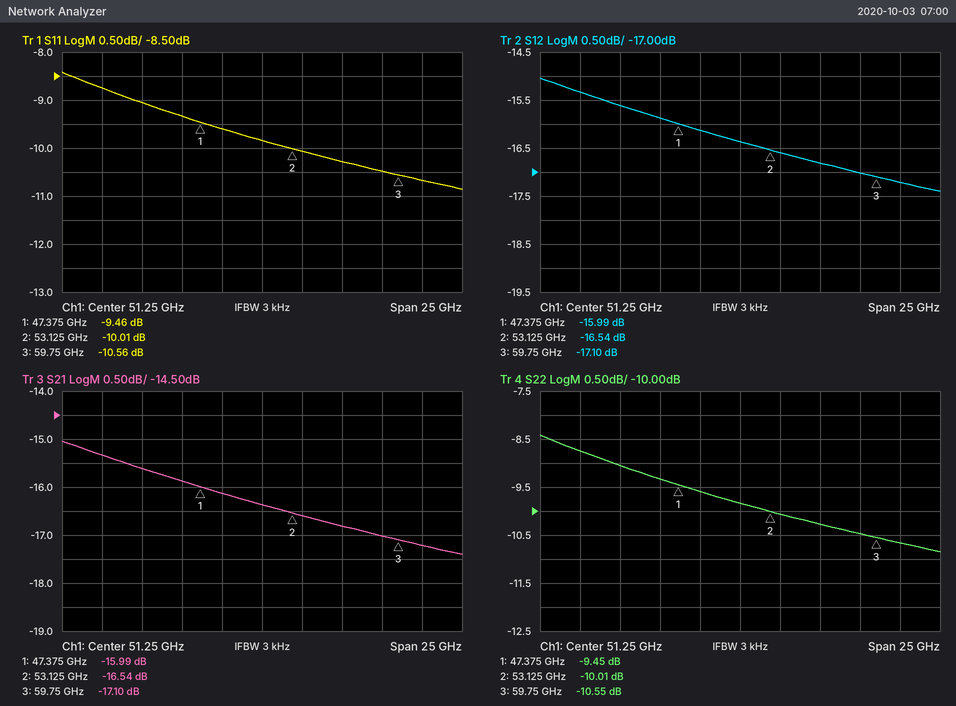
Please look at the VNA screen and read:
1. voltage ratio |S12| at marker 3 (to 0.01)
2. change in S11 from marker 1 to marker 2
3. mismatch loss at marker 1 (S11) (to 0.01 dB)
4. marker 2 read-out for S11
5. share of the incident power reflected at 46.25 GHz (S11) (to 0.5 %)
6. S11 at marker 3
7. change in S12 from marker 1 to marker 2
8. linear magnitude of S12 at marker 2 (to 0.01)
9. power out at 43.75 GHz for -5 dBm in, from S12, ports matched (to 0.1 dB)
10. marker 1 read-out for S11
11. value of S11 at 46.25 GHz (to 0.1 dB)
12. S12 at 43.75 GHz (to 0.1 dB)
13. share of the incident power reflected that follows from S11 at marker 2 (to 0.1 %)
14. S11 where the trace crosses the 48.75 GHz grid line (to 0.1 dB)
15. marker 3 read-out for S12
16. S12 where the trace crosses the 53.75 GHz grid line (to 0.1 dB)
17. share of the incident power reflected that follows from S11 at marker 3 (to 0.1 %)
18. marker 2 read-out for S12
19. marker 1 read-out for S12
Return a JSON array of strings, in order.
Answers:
["0.14", "-0.55 dB", "0.52 dB", "-10.01 dB", "11.5 %", "-10.56 dB", "-0.55 dB", "0.15", "-20.6 dBm", "-9.46 dB", "-9.3 dB", "-15.6 dB", "10.0 %", "-9.6 dB", "-17.10 dB", "-16.6 dB", "8.8 %", "-16.54 dB", "-15.99 dB"]
